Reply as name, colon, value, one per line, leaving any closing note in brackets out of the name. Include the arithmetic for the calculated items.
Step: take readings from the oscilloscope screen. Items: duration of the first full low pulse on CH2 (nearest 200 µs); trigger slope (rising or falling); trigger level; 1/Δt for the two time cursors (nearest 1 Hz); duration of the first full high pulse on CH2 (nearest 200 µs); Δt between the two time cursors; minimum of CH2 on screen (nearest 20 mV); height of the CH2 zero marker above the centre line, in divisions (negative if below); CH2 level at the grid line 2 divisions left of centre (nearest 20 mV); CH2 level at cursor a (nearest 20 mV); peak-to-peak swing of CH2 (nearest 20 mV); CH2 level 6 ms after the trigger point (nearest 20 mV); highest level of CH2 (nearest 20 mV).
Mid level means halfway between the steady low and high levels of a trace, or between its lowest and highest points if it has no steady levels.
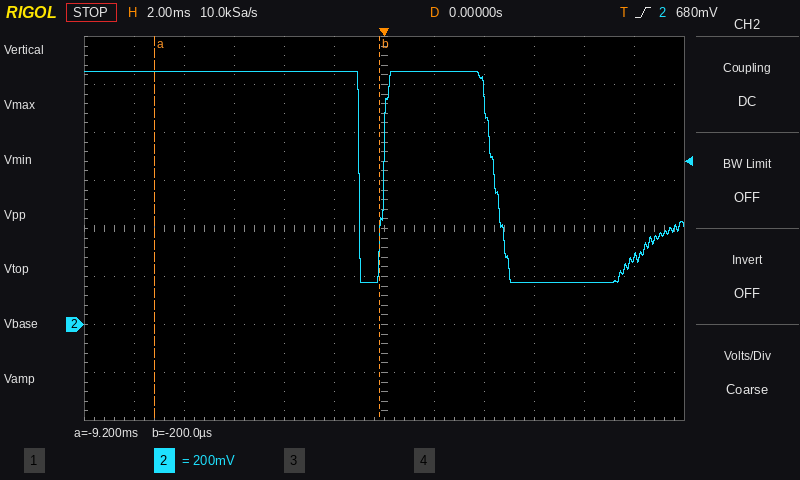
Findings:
duration of the first full low pulse on CH2: 1.0 ms
trigger slope: rising
trigger level: 680 mV
1/Δt for the two time cursors: 1 / 9.0 ms ≈ 111 Hz
duration of the first full high pulse on CH2: 4.4 ms
Δt between the two time cursors: -200 µs − (-9.2 ms) = 9.0 ms
minimum of CH2 on screen: 180 mV
height of the CH2 zero marker above the centre line, in divisions: -2.0 div
CH2 level at the grid line 2 divisions left of centre: 1.06 V
CH2 level at cursor a: 1.06 V
peak-to-peak swing of CH2: 1.06 V − (180 mV) = 880 mV
CH2 level 6 ms after the trigger point: 180 mV
highest level of CH2: 1.06 V
